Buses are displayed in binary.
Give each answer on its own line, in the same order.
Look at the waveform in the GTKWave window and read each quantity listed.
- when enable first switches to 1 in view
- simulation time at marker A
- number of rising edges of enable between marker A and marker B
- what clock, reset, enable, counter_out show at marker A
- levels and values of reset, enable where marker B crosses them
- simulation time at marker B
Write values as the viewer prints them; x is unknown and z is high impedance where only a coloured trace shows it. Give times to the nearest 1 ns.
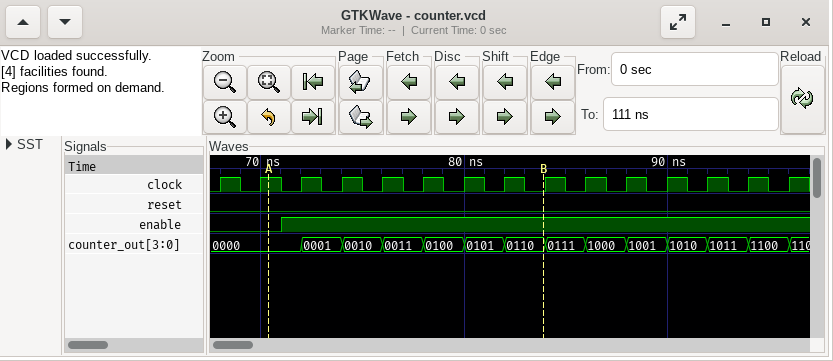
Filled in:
71 ns
70 ns
1
clock=1, reset=0, enable=0, counter_out=0000
reset=0, enable=1
84 ns
